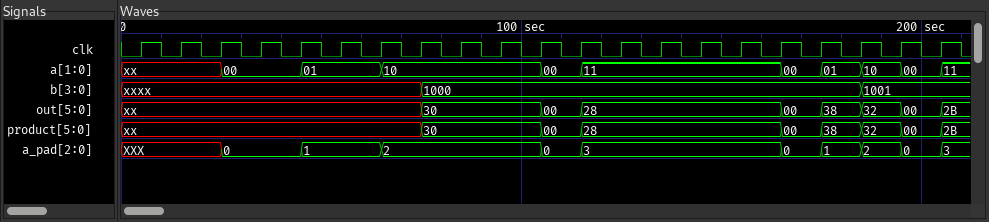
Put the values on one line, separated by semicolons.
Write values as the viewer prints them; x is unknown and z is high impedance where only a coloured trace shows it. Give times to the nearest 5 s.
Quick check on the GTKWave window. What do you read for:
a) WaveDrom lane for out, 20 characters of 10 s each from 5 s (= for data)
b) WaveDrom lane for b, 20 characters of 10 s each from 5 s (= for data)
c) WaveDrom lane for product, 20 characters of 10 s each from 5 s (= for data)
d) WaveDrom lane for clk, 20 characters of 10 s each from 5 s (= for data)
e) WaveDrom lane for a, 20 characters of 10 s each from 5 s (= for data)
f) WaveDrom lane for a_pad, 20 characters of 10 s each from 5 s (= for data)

{name: 'out', wave: 'x......=..==....====', data: '30 00 28 00 38 32 00'}; {name: 'b', wave: 'x......=..........=.', data: '1000 1001'}; {name: 'product', wave: 'x......=..==....====', data: '30 00 28 00 38 32 00'}; {name: 'clk', wave: 'p...................'}; {name: 'a', wave: 'x.=.=.=...==....====', data: '00 01 10 00 11 00 01 10 00'}; {name: 'a_pad', wave: '=.=.=.=...==....====', data: 'XXX 0 1 2 0 3 0 1 2 0'}
